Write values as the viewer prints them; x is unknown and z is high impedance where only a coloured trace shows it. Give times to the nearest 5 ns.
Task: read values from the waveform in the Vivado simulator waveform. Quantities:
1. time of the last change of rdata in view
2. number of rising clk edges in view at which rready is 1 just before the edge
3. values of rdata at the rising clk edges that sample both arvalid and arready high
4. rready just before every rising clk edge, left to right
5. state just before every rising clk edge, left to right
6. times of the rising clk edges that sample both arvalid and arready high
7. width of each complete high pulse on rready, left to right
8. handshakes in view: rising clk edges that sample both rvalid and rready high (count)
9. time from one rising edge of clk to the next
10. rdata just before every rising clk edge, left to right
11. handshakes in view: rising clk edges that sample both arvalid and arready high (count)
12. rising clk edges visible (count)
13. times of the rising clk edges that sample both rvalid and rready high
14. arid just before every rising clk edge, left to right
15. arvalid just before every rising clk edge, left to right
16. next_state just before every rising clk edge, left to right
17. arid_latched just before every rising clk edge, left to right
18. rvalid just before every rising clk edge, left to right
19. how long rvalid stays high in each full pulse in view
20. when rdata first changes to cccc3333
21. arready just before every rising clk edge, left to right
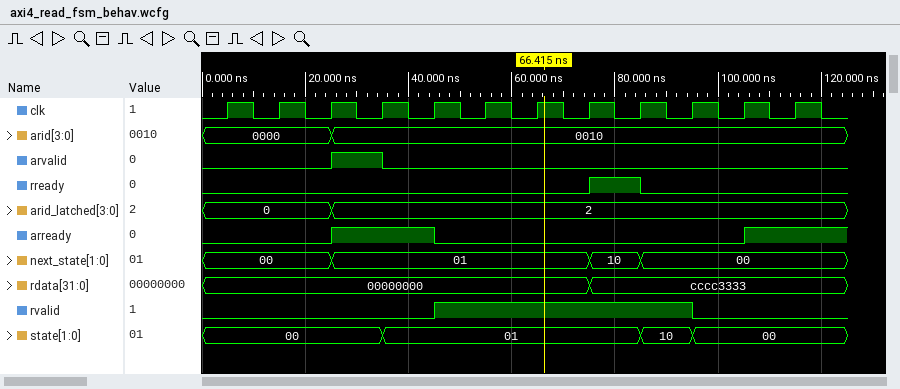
75 ns
1
00000000
0 0 0 0 0 0 0 0 1 0 0 0
00, 00, 00, 00, 01, 01, 01, 01, 01, 10, 00, 00
35 ns
10 ns
1
10 ns
00000000, 00000000, 00000000, 00000000, 00000000, 00000000, 00000000, 00000000, cccc3333, cccc3333, cccc3333, cccc3333
1
12
85 ns
0000, 0000, 0000, 0010, 0010, 0010, 0010, 0010, 0010, 0010, 0010, 0010
0 0 0 1 0 0 0 0 0 0 0 0
00, 00, 00, 01, 01, 01, 01, 01, 10, 00, 00, 00
0, 0, 0, 2, 2, 2, 2, 2, 2, 2, 2, 2
0 0 0 0 0 1 1 1 1 1 0 0
50 ns
75 ns
0 0 0 1 1 0 0 0 0 0 0 1
